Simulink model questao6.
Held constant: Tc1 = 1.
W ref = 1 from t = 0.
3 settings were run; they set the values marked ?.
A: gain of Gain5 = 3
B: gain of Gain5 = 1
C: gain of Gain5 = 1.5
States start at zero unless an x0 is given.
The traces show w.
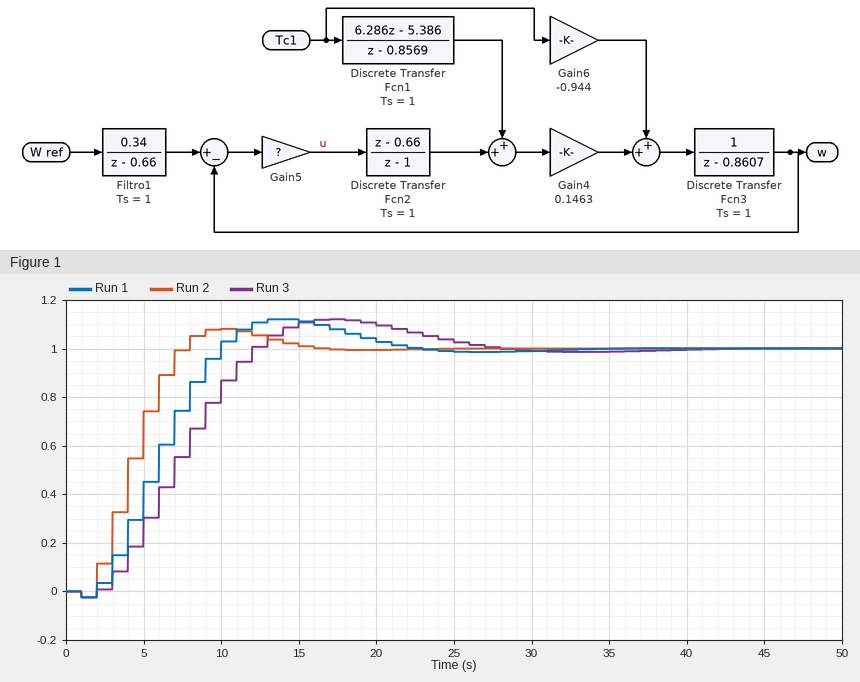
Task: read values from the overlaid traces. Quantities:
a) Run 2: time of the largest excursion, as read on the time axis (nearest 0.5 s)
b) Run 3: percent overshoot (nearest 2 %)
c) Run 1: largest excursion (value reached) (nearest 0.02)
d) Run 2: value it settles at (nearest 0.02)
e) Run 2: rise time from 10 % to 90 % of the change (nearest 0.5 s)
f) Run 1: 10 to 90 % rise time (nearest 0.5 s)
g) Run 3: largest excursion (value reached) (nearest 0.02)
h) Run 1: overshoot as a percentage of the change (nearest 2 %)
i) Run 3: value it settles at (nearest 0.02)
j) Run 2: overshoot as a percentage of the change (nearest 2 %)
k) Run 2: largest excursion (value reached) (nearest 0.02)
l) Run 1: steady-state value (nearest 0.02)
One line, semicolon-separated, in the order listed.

10.0 s; 12 %; 1.12; 1.00; 5.0 s; 6.0 s; 1.12; 12 %; 1.00; 8 %; 1.08; 1.00
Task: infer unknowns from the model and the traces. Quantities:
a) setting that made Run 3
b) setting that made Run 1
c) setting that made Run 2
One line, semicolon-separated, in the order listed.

B; C; A
